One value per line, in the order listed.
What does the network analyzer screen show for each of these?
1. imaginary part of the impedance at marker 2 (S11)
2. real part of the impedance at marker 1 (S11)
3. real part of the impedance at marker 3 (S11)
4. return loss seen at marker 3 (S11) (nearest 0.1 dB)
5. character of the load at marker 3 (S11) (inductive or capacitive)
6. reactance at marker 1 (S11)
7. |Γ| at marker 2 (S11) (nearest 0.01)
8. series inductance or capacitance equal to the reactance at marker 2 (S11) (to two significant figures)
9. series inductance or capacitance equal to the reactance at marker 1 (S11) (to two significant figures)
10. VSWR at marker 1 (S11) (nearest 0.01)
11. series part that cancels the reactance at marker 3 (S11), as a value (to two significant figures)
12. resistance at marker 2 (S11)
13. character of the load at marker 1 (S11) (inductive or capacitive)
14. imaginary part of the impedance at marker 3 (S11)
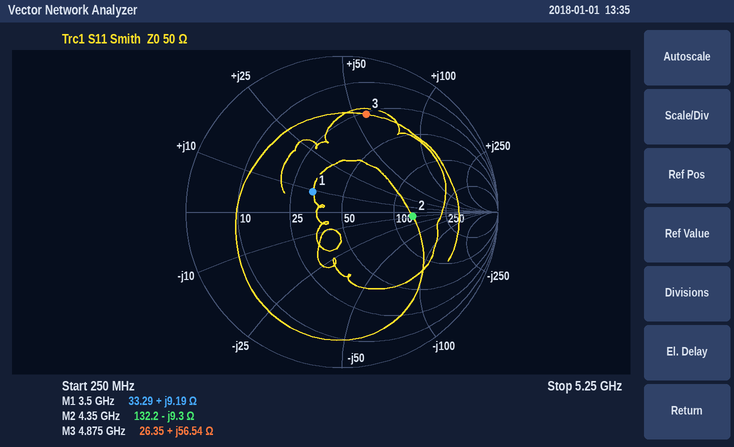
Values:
-9.3 Ω
33.29 Ω
26.35 Ω
3.8 dB
inductive
+9.19 Ω
0.45
3.9 pF
420 pH
1.59
580 fF
132.2 Ω
inductive
+56.54 Ω
